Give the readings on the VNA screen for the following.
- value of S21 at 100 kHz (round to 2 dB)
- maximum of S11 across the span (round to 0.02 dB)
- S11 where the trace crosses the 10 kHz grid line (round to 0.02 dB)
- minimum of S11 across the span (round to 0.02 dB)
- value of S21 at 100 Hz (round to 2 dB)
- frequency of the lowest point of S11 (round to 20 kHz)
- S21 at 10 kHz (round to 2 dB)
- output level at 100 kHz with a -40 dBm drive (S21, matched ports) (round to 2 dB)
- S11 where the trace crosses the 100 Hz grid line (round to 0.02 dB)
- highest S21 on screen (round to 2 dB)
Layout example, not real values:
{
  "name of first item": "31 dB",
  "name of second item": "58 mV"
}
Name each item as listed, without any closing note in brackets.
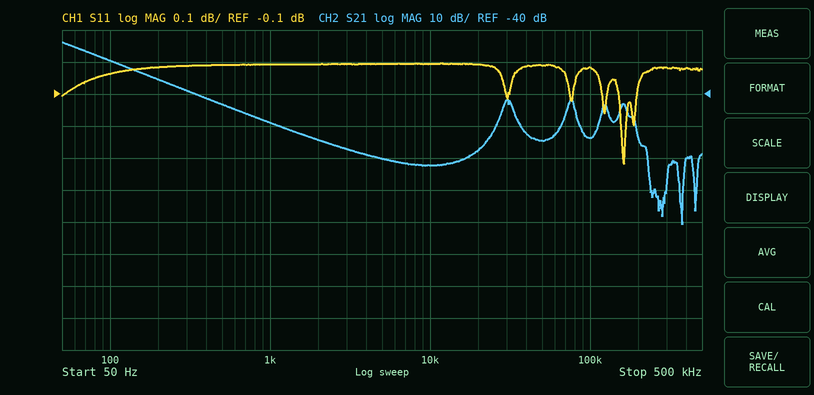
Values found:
{
  "value of S21 at 100 kHz": "-54 dB",
  "maximum of S11 across the span": "0.00 dB",
  "S11 where the trace crosses the 10 kHz grid line": "0.00 dB",
  "minimum of S11 across the span": "-0.32 dB",
  "value of S21 at 100 Hz": "-30 dB",
  "frequency of the lowest point of S11": "160 kHz",
  "S21 at 10 kHz": "-62 dB",
  "output level at 100 kHz with a -40 dBm drive (S21, matched ports)": "-94 dBm",
  "S11 where the trace crosses the 100 Hz grid line": "-0.04 dB",
  "highest S21 on screen": "-24 dB"
}
